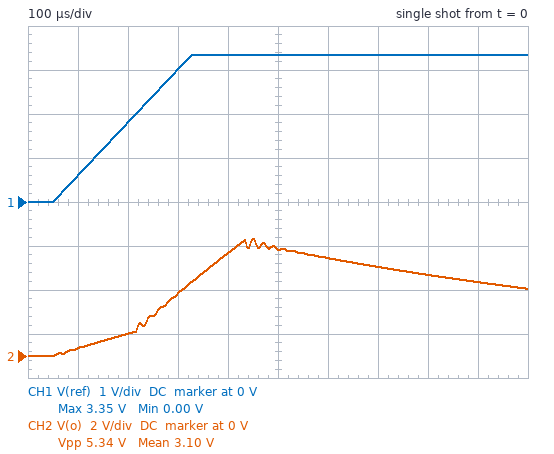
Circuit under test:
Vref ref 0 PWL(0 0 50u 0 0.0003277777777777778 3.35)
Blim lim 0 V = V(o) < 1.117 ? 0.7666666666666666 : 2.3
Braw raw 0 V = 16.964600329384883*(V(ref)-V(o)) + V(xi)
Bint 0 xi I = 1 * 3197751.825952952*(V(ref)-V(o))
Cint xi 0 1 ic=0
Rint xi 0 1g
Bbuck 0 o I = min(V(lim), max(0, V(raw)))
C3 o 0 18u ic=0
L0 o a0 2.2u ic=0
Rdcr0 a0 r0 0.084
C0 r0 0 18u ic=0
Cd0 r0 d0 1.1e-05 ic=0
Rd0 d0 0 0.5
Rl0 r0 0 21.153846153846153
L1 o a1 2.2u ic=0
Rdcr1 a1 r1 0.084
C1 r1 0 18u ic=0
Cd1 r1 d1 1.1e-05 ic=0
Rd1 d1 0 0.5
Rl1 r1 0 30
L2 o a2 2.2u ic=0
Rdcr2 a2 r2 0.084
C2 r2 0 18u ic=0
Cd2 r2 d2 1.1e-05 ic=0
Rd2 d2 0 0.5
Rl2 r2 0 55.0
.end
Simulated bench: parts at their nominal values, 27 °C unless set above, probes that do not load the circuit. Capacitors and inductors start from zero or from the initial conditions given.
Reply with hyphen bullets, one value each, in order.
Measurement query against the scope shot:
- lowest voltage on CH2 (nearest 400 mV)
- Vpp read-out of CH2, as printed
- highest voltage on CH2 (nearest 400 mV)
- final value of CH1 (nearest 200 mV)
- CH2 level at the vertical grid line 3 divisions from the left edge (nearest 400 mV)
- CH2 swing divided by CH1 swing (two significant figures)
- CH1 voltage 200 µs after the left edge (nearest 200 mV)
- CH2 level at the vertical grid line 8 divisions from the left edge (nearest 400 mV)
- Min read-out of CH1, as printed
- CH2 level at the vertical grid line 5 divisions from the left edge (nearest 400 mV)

- 0 V
- 5.34 V
- 5.2 V
- 3.4 V
- 2.8 V
- 1.6
- 1.8 V
- 3.6 V
- 0.00 V
- 4.8 V
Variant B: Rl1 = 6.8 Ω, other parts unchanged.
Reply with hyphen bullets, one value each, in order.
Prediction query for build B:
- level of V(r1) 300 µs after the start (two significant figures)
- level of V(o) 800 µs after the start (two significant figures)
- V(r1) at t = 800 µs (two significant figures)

- 2.3 V
- 3.0 V
- 2.9 V
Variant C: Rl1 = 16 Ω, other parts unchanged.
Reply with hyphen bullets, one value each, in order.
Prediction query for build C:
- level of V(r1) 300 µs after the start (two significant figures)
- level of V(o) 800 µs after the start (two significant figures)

- 2.7 V
- 3.4 V
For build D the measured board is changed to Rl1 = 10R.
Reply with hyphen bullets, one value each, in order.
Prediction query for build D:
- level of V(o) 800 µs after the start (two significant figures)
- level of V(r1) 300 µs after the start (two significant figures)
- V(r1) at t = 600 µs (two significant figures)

- 3.2 V
- 2.5 V
- 4.3 V
